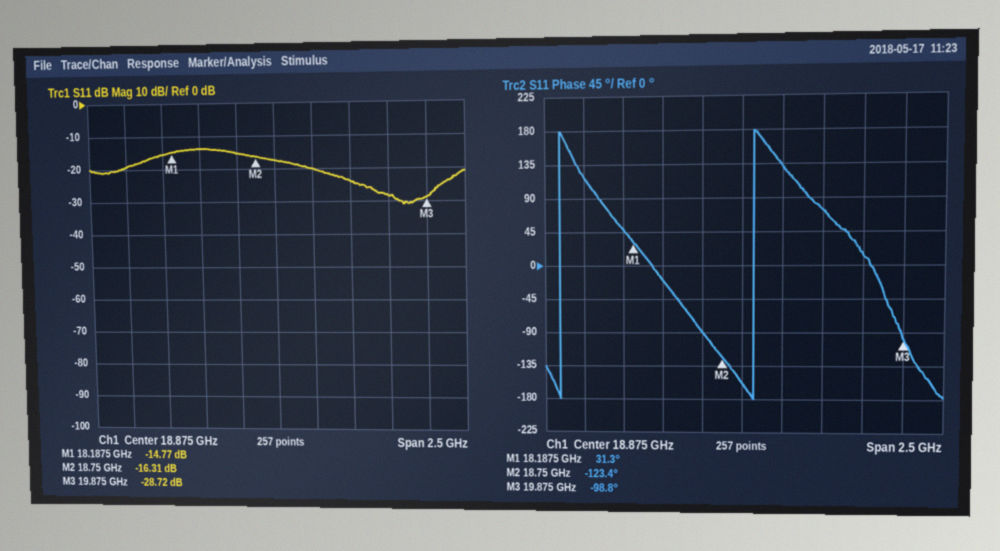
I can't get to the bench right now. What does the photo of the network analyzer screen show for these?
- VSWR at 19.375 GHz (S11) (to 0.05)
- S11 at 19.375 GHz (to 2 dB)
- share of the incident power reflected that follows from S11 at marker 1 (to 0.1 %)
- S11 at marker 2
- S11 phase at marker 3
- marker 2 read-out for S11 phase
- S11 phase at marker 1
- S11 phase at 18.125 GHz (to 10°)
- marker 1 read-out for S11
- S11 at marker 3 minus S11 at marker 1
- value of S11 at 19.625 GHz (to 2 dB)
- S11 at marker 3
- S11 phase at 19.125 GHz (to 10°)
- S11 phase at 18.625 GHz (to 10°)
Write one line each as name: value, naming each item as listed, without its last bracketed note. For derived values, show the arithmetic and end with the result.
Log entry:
VSWR at 19.375 GHz (S11): |Γ| = 10^(-24/20) = 0.0631; VSWR = (1 + 0.0631)/(1 − 0.0631) ≈ 1.13, so 1.15 to the nearest 0.05
S11 at 19.375 GHz: -24 dB
share of the incident power reflected that follows from S11 at marker 1: 10^(-14.77/10) ≈ 3.3 %
S11 at marker 2: -16.31 dB
S11 phase at marker 3: -98.8°
marker 2 read-out for S11 phase: -123.4°
S11 phase at marker 1: 31.3°
S11 phase at 18.125 GHz: 50°
marker 1 read-out for S11: -14.77 dB
S11 at marker 3 minus S11 at marker 1: -28.72 − (-14.77) = -13.95 dB
value of S11 at 19.625 GHz: -28 dB
S11 at marker 3: -28.72 dB
S11 phase at 19.125 GHz: 130°
S11 phase at 18.625 GHz: -90°
